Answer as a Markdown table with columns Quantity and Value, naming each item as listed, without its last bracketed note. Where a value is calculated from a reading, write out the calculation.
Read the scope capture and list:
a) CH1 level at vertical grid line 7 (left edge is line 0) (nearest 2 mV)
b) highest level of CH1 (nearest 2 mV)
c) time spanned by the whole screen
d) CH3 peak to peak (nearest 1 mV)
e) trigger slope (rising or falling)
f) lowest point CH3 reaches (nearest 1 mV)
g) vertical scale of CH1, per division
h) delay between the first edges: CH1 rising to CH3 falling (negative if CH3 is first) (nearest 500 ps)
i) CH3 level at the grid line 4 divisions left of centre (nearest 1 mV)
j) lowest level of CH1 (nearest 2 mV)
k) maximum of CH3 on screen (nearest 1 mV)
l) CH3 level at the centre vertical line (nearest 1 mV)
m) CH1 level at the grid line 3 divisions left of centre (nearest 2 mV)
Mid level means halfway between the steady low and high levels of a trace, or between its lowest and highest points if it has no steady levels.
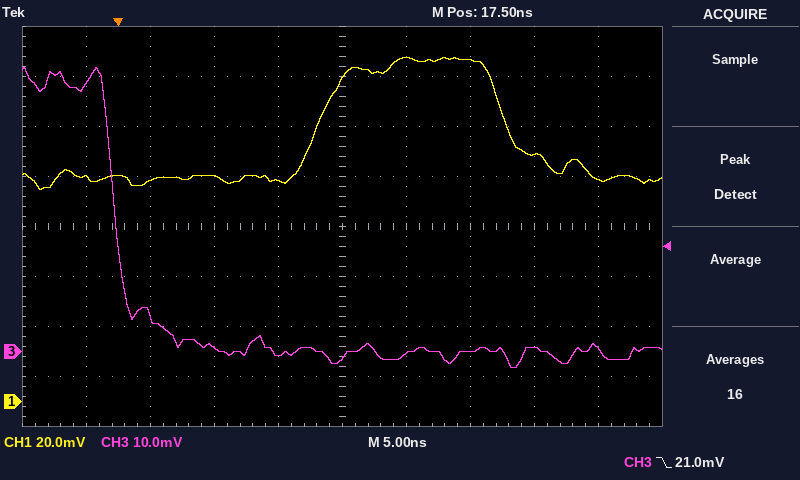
| Quantity | Value |
|---|---|
| CH1 level at vertical grid line 7 (left edge is line 0) | 136 mV |
| highest level of CH1 | 138 mV |
| time spanned by the whole screen | 50 ns |
| CH3 peak to peak | 57 mV − (-3 mV) = 60 mV |
| trigger slope | falling |
| lowest point CH3 reaches | -3 mV |
| vertical scale of CH1, per division | 20 mV |
| delay between the first edges: CH1 rising to CH3 falling (negative if CH3 is first) | -16.0 ns |
| CH3 level at the grid line 4 divisions left of centre | 54 mV |
| lowest level of CH1 | 84 mV |
| maximum of CH3 on screen | 57 mV |
| CH3 level at the centre vertical line | -1 mV |
| CH1 level at the grid line 3 divisions left of centre | 88 mV |
